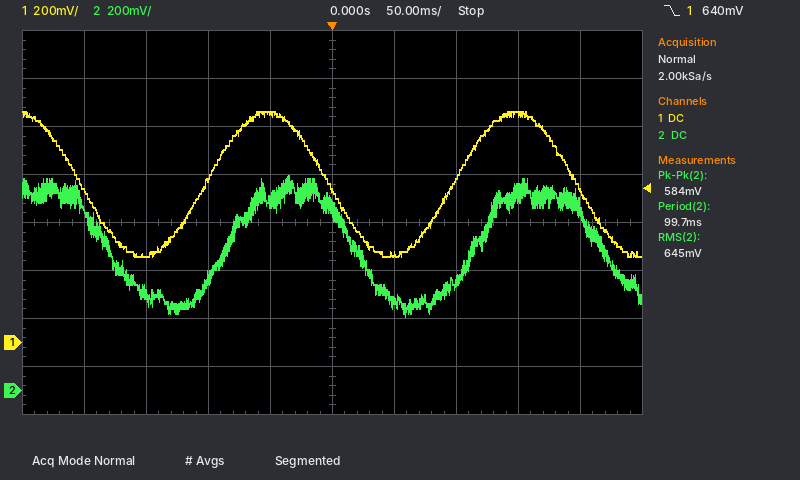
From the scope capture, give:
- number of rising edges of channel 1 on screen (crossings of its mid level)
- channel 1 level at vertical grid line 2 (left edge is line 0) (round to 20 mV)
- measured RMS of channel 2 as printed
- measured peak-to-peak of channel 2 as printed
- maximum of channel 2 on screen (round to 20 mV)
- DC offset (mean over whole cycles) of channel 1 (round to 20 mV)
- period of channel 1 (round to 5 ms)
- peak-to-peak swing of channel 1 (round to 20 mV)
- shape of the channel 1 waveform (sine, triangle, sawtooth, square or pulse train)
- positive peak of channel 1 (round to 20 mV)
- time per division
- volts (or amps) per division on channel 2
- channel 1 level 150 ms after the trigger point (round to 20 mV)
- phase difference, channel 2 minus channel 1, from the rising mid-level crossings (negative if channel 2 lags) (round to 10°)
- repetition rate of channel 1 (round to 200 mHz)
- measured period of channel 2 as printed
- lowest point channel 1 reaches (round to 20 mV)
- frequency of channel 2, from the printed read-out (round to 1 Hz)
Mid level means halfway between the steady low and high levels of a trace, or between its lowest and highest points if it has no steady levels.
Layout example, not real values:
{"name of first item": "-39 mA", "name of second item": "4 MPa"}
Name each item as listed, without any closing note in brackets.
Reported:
{"number of rising edges of channel 1 on screen": "2", "channel 1 level at vertical grid line 2 (left edge is line 0)": "360 mV", "measured RMS of channel 2 as printed": "645 mV", "measured peak-to-peak of channel 2 as printed": "584 mV", "maximum of channel 2 on screen": "900 mV", "DC offset (mean over whole cycles) of channel 1": "660 mV", "period of channel 1": "200 ms", "peak-to-peak swing of channel 1": "600 mV", "shape of the channel 1 waveform": "sine", "positive peak of channel 1": "960 mV", "time per division": "50 ms", "volts (or amps) per division on channel 2": "200 mV", "channel 1 level 150 ms after the trigger point": "960 mV", "phase difference, channel 2 minus channel 1, from the rising mid-level crossings (negative if channel 2 lags)": "-30°", "repetition rate of channel 1": "5.0 Hz", "measured period of channel 2 as printed": "99.7 ms", "lowest point channel 1 reaches": "360 mV", "frequency of channel 2, from the printed read-out": "10 Hz"}
